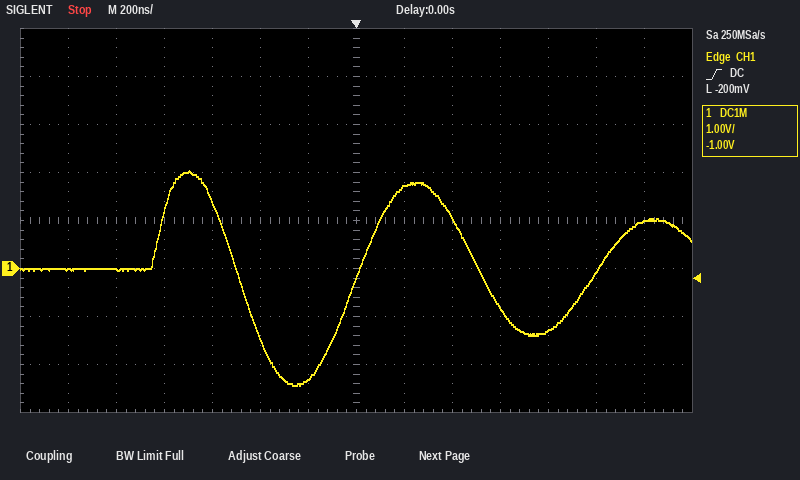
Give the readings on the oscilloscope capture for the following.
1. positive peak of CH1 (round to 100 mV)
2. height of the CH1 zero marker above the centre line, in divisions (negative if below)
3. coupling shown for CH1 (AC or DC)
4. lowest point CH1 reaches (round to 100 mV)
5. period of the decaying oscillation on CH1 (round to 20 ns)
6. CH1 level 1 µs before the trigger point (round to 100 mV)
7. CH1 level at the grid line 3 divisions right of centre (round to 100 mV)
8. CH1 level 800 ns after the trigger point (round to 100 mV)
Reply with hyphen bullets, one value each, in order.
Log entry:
- 2.0 V
- -1.0 div
- DC
- -2.4 V
- 980 ns
- 0.0 V
- -800 mV
- -1.3 V
